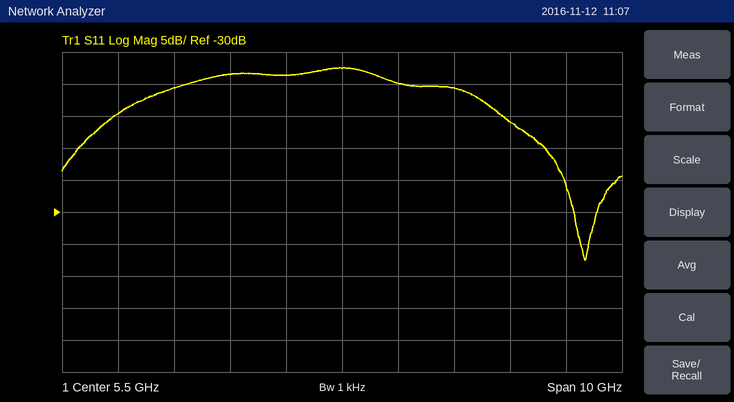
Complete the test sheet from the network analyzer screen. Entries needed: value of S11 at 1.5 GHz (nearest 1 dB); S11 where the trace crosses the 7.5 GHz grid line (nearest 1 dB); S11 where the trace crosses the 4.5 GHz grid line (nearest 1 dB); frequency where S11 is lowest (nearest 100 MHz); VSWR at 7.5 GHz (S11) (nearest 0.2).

-15 dB
-11 dB
-9 dB
9.8 GHz
1.8
